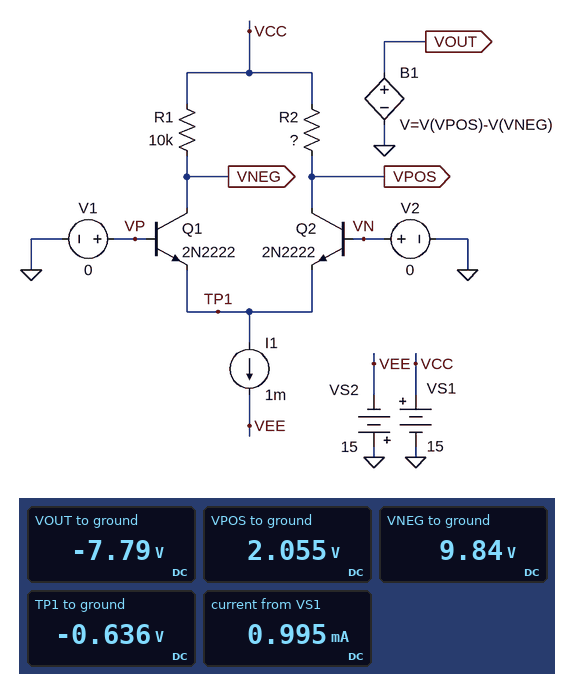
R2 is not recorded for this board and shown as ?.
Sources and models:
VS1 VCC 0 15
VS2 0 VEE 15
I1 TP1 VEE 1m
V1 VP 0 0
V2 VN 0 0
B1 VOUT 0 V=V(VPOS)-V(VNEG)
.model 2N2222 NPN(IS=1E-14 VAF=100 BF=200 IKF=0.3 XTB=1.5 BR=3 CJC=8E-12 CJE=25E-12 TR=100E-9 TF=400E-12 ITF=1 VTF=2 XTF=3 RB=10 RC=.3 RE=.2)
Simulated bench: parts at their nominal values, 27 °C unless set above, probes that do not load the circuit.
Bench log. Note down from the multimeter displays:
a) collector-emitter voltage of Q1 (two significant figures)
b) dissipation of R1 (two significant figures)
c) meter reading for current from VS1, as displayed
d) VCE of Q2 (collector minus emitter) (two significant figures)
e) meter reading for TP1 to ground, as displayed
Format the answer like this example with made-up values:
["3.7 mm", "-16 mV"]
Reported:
["10 V", "2.7 mW", "0.995 mA", "2.7 V", "-0.636 V"]
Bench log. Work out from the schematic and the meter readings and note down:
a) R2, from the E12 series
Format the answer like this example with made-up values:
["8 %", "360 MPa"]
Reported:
["27 kΩ"]
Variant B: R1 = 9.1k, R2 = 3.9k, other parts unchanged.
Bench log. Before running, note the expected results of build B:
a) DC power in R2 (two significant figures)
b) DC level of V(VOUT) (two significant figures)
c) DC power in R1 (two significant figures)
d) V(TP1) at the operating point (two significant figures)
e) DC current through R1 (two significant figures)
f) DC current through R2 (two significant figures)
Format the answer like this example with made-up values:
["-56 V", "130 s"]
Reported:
["990 µW", "2.5 V", "2.2 mW", "-630 mV", "490 µA", "500 µA"]
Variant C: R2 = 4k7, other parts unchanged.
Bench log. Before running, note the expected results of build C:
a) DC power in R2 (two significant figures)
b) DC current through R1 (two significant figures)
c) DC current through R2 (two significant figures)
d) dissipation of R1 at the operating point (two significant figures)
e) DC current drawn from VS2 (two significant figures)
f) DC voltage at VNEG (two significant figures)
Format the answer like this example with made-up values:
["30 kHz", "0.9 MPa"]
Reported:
["1.2 mW", "490 µA", "500 µA", "2.4 mW", "1.0 mA", "10 V"]
